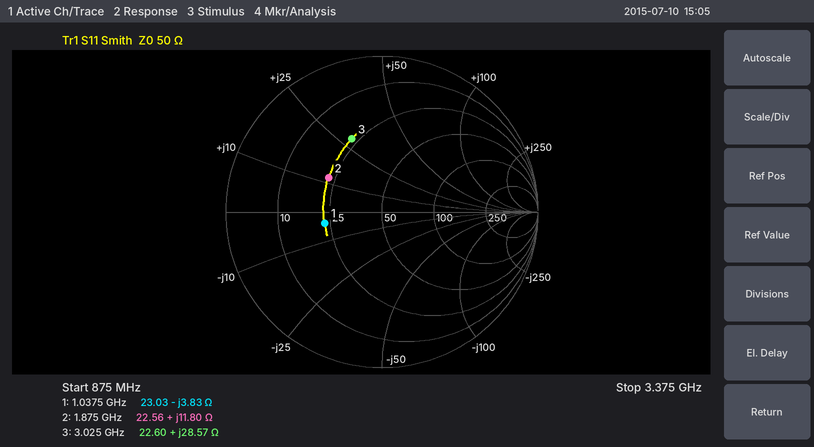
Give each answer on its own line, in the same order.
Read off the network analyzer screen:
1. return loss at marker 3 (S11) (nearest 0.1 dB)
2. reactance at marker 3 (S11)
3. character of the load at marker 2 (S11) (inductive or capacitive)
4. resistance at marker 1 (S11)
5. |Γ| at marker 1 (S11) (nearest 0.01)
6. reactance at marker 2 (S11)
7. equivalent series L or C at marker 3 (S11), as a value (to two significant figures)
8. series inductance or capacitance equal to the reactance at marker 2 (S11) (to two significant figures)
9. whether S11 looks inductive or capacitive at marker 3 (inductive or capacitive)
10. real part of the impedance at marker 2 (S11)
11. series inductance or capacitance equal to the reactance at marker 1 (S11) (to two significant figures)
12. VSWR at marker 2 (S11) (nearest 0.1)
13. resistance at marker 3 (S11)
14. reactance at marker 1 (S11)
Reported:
5.9 dB
+28.57 Ω
inductive
23.03 Ω
0.37
+11.80 Ω
1.5 nH
1.0 nH
inductive
22.56 Ω
40 pF
2.4
22.60 Ω
-3.83 Ω
